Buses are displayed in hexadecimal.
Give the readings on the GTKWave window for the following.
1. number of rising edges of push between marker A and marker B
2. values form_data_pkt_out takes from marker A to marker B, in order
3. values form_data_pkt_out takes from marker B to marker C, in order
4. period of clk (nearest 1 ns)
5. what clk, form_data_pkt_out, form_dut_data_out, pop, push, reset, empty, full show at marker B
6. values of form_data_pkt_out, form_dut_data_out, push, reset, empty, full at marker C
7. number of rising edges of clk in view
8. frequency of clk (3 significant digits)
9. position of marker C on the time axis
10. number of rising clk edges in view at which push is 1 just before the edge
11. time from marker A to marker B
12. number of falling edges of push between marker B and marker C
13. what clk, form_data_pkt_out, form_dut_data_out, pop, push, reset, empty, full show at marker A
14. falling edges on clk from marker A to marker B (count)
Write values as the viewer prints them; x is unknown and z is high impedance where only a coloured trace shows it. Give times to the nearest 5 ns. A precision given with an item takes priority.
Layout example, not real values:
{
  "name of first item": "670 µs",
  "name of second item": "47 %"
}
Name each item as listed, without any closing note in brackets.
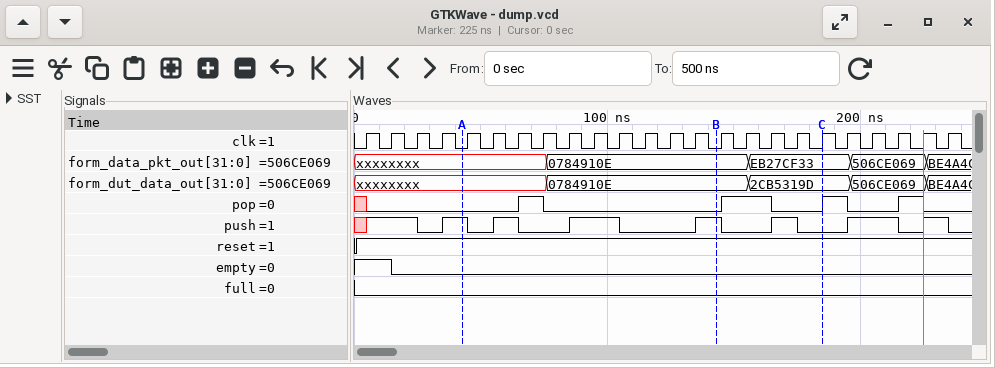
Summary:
{
  "number of rising edges of push between marker A and marker B": "3",
  "values form_data_pkt_out takes from marker A to marker B, in order": "xxxxxxxx, 0784910E",
  "values form_data_pkt_out takes from marker B to marker C, in order": "0784910E, EB27CF33",
  "period of clk": "10 ns",
  "what clk, form_data_pkt_out, form_dut_data_out, pop, push, reset, empty, full show at marker B": "clk=0, form_data_pkt_out=0784910E, form_dut_data_out=0784910E, pop=0, push=1, reset=1, empty=0, full=0",
  "values of form_data_pkt_out, form_dut_data_out, push, reset, empty, full at marker C": "form_data_pkt_out=EB27CF33, form_dut_data_out=2CB5319D, push=0, reset=1, empty=0, full=0",
  "number of rising edges of clk in view": "24",
  "frequency of clk": "100 MHz",
  "position of marker C on the time axis": "185 ns",
  "number of rising clk edges in view at which push is 1 just before the edge": "11",
  "time from marker A to marker B": "100 ns",
  "number of falling edges of push between marker B and marker C": "2",
  "what clk, form_data_pkt_out, form_dut_data_out, pop, push, reset, empty, full show at marker A": "clk=0, form_data_pkt_out=xxxxxxxx, form_dut_data_out=xxxxxxxx, pop=0, push=1, reset=1, empty=0, full=0",
  "falling edges on clk from marker A to marker B": "10"
}
